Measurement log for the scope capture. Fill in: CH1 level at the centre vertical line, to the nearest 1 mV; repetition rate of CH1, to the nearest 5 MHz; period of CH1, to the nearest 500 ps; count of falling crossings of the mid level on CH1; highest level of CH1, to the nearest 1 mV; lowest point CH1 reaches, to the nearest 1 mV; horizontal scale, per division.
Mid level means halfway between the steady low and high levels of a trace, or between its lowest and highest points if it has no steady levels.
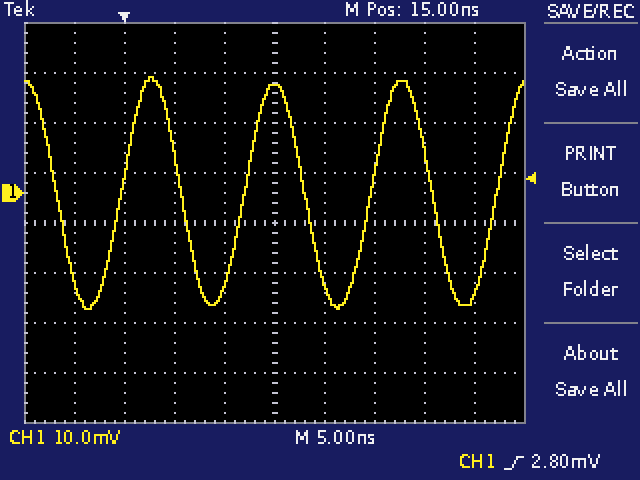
22 mV
80 MHz
12.5 ns
4
23 mV
-23 mV
5 ns
